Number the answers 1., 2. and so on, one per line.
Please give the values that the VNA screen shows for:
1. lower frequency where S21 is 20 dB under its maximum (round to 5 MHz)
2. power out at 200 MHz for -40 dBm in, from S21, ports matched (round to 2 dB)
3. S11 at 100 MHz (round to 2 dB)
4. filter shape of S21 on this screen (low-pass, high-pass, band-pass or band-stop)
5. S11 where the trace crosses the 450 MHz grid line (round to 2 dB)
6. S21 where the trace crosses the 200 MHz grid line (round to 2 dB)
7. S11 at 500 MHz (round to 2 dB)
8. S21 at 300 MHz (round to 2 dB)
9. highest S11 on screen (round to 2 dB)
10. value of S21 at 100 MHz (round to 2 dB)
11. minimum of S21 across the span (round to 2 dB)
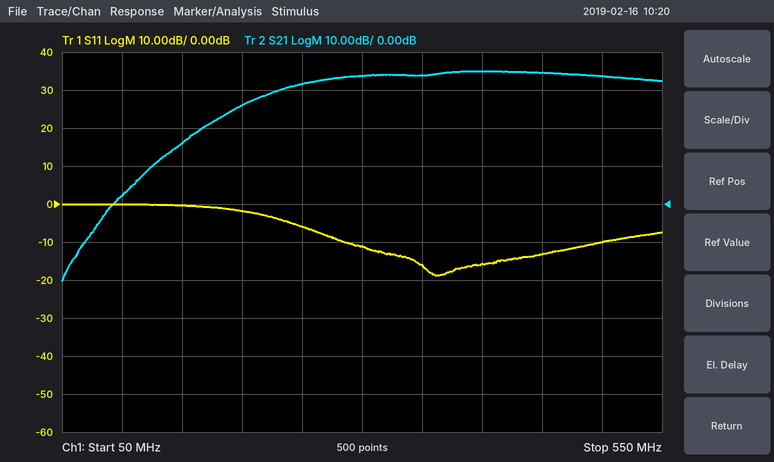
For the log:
1. 145 MHz
2. -14 dBm
3. 0 dB
4. high-pass
5. -14 dB
6. 26 dB
7. -10 dB
8. 34 dB
9. 0 dB
10. 2 dB
11. -20 dB
